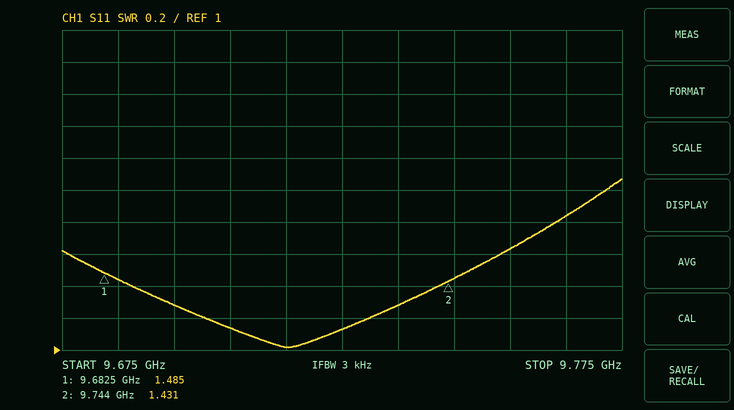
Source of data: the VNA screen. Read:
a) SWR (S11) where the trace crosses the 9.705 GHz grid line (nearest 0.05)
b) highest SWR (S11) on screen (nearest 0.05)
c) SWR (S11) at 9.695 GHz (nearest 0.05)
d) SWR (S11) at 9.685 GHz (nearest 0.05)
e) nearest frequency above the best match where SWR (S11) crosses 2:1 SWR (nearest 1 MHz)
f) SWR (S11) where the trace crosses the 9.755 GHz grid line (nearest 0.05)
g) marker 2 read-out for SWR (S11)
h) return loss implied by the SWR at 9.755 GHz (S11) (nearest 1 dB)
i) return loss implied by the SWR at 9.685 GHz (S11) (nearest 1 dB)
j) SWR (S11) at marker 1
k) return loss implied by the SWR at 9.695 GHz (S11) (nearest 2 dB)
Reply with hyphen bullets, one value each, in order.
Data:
- 1.15
- 2.05
- 1.30
- 1.45
- 9.772 GHz
- 1.65
- 1.431
- 12 dB
- 15 dB
- 1.485
- 18 dB
